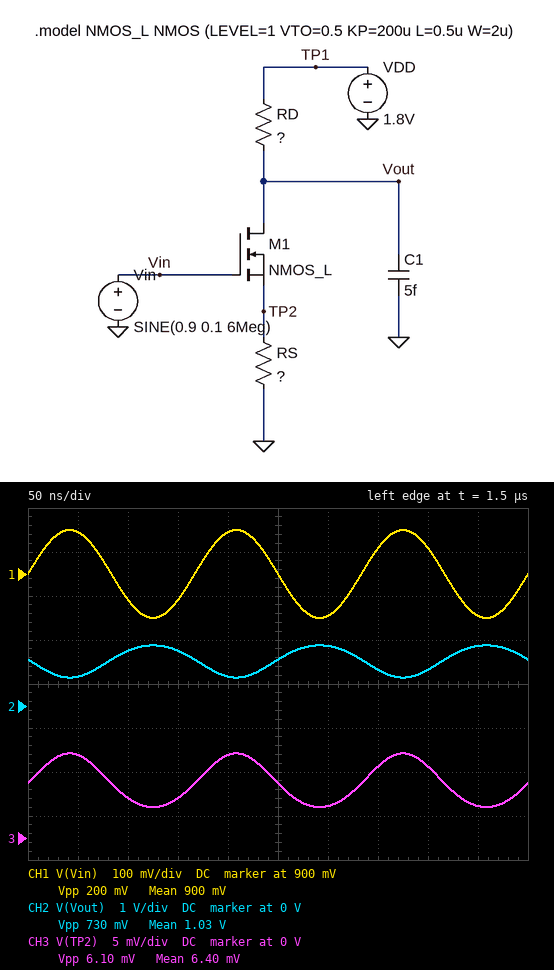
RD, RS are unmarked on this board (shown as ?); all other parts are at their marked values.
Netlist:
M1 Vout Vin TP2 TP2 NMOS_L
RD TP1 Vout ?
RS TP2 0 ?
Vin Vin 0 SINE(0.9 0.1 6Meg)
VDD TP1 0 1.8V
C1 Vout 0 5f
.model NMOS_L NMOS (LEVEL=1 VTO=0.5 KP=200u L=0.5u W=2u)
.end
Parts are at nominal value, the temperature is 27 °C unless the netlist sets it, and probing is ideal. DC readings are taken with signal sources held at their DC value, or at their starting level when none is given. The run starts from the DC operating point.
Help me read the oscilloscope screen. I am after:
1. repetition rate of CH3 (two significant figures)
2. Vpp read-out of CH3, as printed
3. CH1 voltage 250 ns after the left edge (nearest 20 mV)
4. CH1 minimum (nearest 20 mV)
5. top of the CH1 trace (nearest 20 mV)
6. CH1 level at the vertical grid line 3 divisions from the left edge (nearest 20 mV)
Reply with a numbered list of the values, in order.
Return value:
1. 6.0 MHz
2. 6.10 mV
3. 900 mV
4. 800 mV
5. 1.00 V
6. 840 mV
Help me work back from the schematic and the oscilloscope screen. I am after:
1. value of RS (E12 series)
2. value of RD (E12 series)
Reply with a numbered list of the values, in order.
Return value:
1. 100 Ω
2. 12 kΩ
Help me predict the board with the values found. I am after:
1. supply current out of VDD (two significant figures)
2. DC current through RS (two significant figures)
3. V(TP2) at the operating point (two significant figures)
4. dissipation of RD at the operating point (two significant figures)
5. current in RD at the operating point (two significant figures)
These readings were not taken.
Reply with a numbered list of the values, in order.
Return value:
1. 62 µA
2. 62 µA
3. 6.2 mV
4. 46 µW
5. 62 µA
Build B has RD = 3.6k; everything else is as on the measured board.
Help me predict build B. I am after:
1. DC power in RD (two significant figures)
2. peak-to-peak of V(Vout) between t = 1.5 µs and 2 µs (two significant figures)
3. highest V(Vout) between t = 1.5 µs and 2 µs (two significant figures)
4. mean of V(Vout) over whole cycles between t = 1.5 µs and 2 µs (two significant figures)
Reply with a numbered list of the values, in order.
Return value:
1. 14 µW
2. 220 mV
3. 1.7 V
4. 1.6 V
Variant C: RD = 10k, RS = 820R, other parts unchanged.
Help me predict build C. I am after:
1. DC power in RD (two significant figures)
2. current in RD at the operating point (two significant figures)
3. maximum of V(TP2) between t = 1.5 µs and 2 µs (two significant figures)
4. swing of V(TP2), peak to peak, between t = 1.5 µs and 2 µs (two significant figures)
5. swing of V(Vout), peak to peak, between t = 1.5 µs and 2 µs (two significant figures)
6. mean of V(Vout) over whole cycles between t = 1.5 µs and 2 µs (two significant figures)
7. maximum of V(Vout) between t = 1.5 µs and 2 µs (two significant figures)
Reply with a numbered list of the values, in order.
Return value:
1. 26 µW
2. 51 µA
3. 63 mV
4. 38 mV
5. 460 mV
6. 1.3 V
7. 1.5 V
